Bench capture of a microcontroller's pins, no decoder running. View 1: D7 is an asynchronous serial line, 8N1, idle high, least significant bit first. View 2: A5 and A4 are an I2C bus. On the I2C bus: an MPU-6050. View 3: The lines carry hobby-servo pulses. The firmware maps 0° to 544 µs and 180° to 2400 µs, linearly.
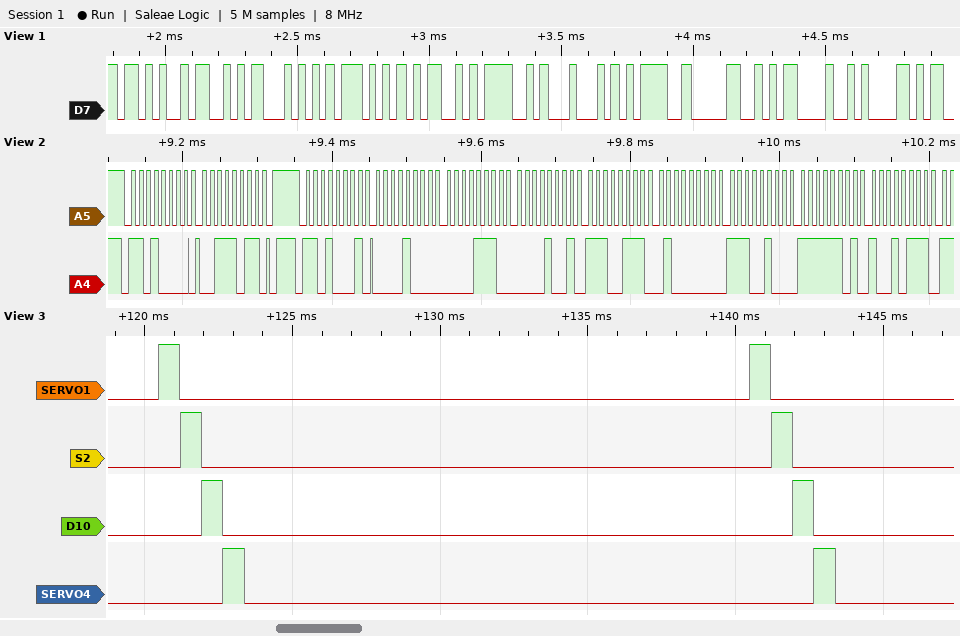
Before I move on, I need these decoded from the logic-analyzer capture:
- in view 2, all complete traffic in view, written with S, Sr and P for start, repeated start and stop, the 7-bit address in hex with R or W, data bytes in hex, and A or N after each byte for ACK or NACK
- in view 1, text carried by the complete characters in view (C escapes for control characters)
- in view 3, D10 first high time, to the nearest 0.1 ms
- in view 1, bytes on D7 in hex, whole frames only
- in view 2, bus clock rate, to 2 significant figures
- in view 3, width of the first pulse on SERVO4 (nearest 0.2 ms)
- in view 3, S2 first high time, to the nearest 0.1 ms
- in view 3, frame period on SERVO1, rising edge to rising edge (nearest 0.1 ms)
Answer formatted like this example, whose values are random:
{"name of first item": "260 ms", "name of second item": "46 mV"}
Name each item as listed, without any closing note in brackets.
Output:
{"in view 2, all complete traffic in view, written with S, Sr and P for start, repeated start and stop, the 7-bit address in hex with R or W, data bytes in hex, and A or N after each byte for ACK or NACK": "S 68W A 3B A P S 68R A 08 A 0E A 09 A E7 A 40 A E4 A FD A 97 A", "in view 1, text carried by the complete characters in view": "\"+STWMOD=0\\r\\n\"", "in view 3, D10 first high time, to the nearest 0.1 ms": "0.7 ms", "in view 1, bytes on D7 in hex, whole frames only": "2B 53 54 57 4D 4F 44 3D 30 0D 0A", "in view 2, bus clock rate, to 2 significant figures": "100 kHz", "in view 3, width of the first pulse on SERVO4": "0.8 ms", "in view 3, S2 first high time, to the nearest 0.1 ms": "0.7 ms", "in view 3, frame period on SERVO1, rising edge to rising edge": "20.0 ms"}
